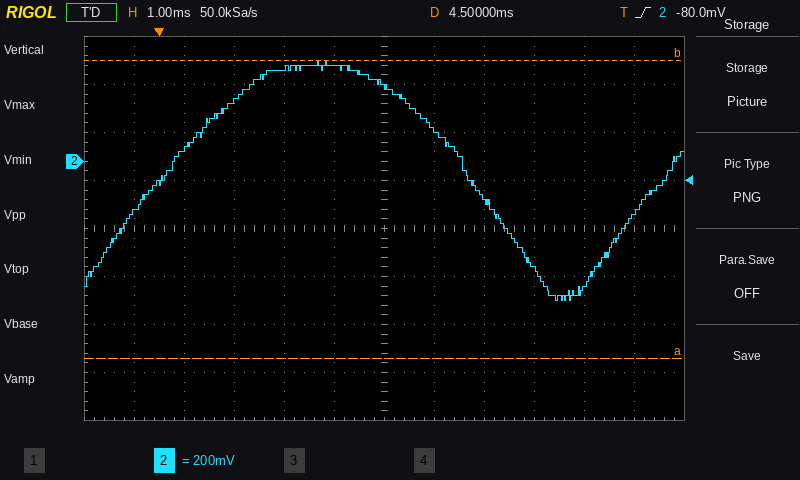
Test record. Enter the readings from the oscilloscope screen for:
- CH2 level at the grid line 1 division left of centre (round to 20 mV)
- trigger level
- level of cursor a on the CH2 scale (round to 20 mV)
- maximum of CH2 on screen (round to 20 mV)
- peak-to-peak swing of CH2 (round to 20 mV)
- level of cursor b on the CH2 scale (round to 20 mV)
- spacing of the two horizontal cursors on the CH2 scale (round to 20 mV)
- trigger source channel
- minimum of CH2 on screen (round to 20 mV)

400 mV
-80.0 mV
-820 mV
420 mV
1.00 V
420 mV
1.24 V
CH2
-580 mV
